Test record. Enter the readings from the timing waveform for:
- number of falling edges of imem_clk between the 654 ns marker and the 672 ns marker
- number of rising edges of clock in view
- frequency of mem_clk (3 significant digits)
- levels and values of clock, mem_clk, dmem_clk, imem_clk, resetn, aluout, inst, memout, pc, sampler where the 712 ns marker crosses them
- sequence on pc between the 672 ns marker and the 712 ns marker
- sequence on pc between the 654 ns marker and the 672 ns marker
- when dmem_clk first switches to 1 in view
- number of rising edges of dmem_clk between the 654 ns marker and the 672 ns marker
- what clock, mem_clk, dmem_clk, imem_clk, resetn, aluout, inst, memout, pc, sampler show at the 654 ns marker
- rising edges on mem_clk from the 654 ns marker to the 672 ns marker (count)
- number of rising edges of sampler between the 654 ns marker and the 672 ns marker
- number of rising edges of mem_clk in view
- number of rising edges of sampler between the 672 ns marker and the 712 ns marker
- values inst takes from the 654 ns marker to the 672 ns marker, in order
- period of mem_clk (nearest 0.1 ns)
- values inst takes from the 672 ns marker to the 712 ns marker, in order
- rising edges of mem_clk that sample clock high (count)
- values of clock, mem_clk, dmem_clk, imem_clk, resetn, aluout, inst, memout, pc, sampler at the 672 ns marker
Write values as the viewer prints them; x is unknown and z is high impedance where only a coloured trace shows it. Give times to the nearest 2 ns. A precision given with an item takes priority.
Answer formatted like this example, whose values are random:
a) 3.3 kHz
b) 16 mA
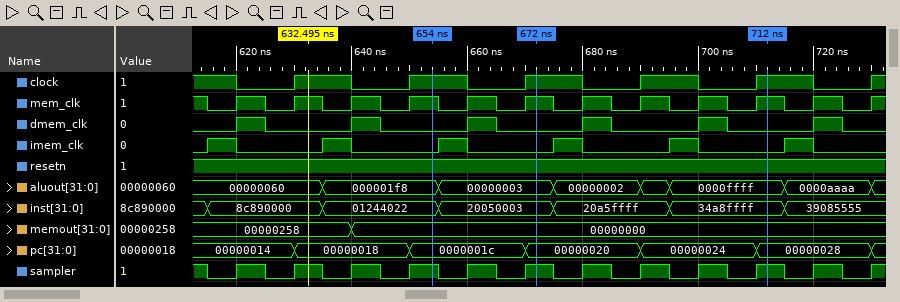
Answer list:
a) 1
b) 6
c) 100 MHz
d) clock=1, mem_clk=1, dmem_clk=0, imem_clk=0, resetn=1, aluout=0000ffff, inst=34a8ffff, memout=00000000, pc=00000028, sampler=1
e) 00000020, 00000024, 00000028
f) 0000001c, 00000020
g) 620 ns
h) 1
i) clock=1, mem_clk=1, dmem_clk=0, imem_clk=0, resetn=1, aluout=000001f8, inst=01244022, memout=00000000, pc=0000001c, sampler=1
j) 2
k) 2
l) 12
m) 4
n) 01244022, 20050003
o) 10 ns
p) 20050003, 20a5ffff, 34a8ffff
q) 6
r) clock=1, mem_clk=1, dmem_clk=0, imem_clk=0, resetn=1, aluout=00000003, inst=20050003, memout=00000000, pc=00000020, sampler=1
